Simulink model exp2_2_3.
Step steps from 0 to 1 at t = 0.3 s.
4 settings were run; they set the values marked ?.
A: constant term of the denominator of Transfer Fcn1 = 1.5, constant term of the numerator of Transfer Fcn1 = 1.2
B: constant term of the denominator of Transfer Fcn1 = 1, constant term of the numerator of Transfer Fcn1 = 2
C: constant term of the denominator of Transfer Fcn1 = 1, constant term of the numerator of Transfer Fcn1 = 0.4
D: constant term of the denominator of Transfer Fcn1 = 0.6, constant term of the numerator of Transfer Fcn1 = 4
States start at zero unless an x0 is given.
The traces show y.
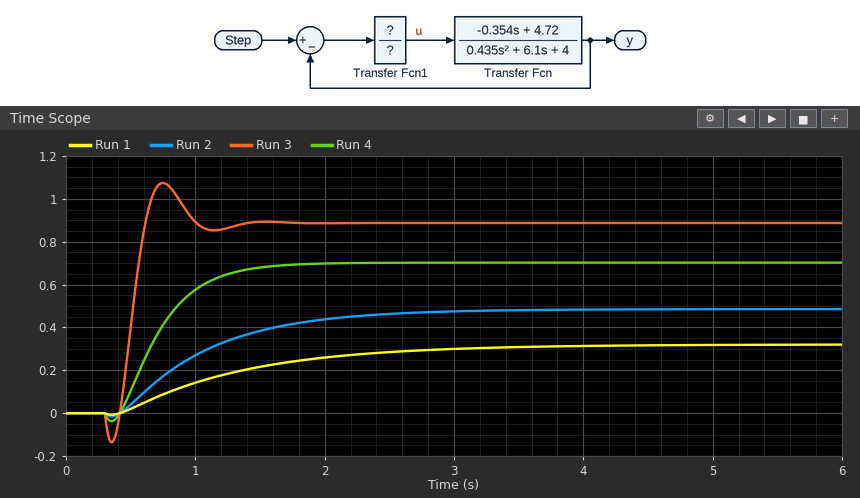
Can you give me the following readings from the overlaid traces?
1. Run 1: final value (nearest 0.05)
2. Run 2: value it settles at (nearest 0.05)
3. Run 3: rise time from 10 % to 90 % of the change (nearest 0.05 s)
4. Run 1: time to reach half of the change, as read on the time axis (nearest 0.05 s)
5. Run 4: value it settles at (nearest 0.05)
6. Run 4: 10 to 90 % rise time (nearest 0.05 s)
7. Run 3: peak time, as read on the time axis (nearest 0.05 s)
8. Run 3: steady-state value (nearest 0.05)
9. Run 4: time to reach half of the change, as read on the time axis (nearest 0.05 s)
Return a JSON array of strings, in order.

["0.30", "0.50", "0.15 s", "1.10 s", "0.70", "0.70 s", "0.75 s", "0.90", "0.70 s"]
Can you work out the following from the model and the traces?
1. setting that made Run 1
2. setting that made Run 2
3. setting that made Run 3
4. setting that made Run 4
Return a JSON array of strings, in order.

["C", "A", "D", "B"]
